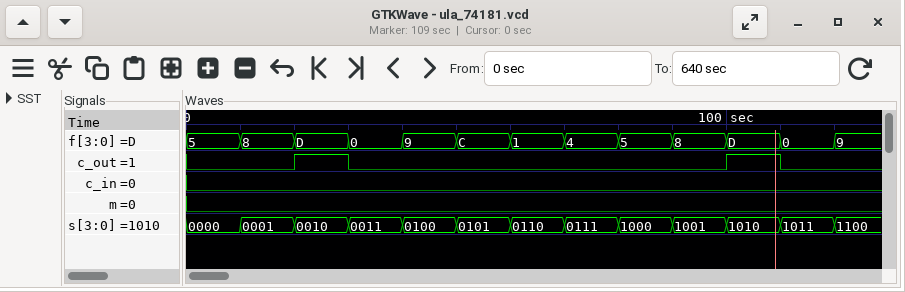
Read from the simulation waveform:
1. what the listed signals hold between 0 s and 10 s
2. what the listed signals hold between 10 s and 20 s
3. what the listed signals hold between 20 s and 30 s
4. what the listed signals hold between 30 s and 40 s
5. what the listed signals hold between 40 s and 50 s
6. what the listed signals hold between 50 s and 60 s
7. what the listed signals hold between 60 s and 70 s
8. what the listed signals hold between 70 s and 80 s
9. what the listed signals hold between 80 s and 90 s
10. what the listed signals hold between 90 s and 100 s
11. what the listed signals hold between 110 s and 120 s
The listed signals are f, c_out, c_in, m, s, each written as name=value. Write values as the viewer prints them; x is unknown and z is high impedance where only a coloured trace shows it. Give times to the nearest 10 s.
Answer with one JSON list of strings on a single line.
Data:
["f=5, c_out=0, c_in=0, m=0, s=0000", "f=8, c_out=0, c_in=0, m=0, s=0001", "f=D, c_out=1, c_in=0, m=0, s=0010", "f=0, c_out=0, c_in=0, m=0, s=0011", "f=9, c_out=0, c_in=0, m=0, s=0100", "f=C, c_out=0, c_in=0, m=0, s=0101", "f=1, c_out=0, c_in=0, m=0, s=0110", "f=4, c_out=0, c_in=0, m=0, s=0111", "f=5, c_out=0, c_in=0, m=0, s=1000", "f=8, c_out=0, c_in=0, m=0, s=1001", "f=0, c_out=0, c_in=0, m=0, s=1011"]
